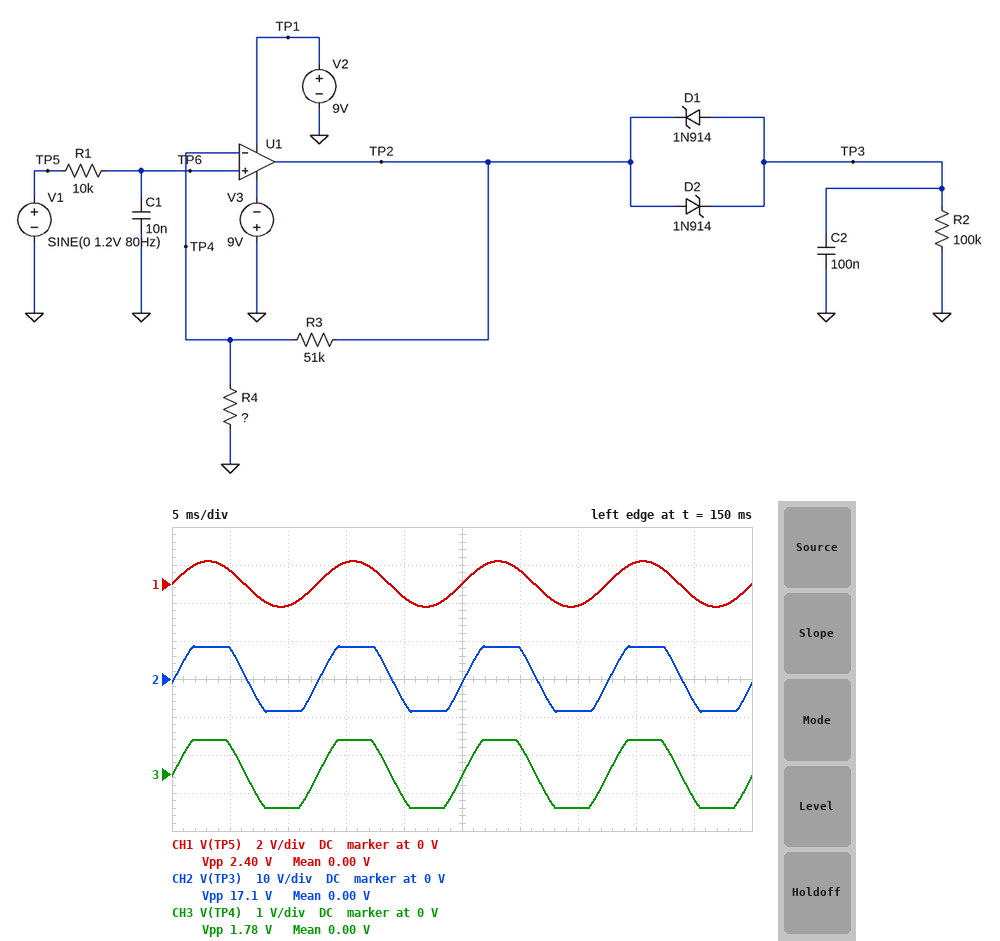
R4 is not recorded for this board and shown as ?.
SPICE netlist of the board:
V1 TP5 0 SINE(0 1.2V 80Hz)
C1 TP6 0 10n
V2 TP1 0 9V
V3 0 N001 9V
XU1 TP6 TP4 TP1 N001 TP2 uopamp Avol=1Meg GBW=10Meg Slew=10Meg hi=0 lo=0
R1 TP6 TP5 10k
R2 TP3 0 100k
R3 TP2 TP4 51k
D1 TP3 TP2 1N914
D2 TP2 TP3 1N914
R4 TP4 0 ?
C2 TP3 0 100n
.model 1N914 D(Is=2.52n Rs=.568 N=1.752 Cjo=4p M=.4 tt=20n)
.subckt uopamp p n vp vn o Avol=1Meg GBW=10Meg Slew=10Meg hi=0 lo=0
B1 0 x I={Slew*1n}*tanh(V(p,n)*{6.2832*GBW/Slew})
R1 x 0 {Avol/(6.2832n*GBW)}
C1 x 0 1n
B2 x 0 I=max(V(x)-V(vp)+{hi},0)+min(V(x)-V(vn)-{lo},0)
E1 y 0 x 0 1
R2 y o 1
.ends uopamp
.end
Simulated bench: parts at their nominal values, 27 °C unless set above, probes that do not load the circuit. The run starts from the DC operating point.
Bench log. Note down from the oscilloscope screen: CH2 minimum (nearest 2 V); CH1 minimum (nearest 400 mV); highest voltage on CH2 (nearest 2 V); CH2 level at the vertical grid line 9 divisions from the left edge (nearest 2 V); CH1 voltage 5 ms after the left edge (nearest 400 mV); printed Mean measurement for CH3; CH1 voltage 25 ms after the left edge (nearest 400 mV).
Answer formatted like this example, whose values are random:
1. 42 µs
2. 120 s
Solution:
1. -8 V
2. -1.2 V
3. 8 V
4. -6 V
5. 800 mV
6. 0.00 V
7. 0 V
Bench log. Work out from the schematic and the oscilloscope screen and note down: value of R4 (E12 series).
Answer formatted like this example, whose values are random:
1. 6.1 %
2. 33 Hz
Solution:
1. 5.6 kΩ
